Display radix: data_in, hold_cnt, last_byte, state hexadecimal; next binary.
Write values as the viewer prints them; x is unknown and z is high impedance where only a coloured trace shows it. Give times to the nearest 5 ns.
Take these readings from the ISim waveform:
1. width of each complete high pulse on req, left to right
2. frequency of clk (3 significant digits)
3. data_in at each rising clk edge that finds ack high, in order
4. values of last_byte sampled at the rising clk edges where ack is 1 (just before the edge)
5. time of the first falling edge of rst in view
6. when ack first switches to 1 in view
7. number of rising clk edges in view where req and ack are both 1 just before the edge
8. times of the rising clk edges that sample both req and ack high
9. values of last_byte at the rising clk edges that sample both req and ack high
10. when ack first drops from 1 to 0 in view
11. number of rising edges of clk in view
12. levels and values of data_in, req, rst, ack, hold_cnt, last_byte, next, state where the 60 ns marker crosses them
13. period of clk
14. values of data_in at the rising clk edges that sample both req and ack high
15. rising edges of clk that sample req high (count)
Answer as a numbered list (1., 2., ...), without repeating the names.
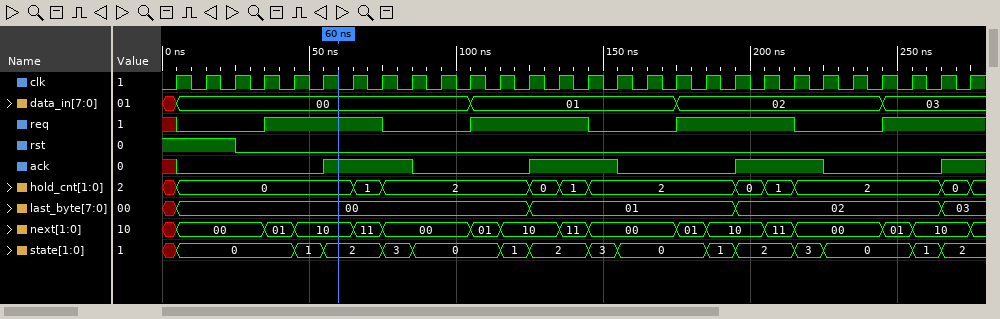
1. 40 ns, 40 ns, 40 ns
2. 100 MHz
3. 00, 00, 00, 01, 01, 01, 02, 02, 02, 03
4. 00, 00, 00, 01, 01, 01, 02, 02, 02, 03
5. 25 ns
6. 55 ns
7. 7
8. 65 ns, 75 ns, 135 ns, 145 ns, 205 ns, 215 ns, 275 ns
9. 00, 00, 01, 01, 02, 02, 03
10. 85 ns
11. 28
12. data_in=00, req=1, rst=0, ack=1, hold_cnt=0, last_byte=00, next=10, state=2
13. 10 ns
14. 00, 00, 01, 01, 02, 02, 03
15. 15
